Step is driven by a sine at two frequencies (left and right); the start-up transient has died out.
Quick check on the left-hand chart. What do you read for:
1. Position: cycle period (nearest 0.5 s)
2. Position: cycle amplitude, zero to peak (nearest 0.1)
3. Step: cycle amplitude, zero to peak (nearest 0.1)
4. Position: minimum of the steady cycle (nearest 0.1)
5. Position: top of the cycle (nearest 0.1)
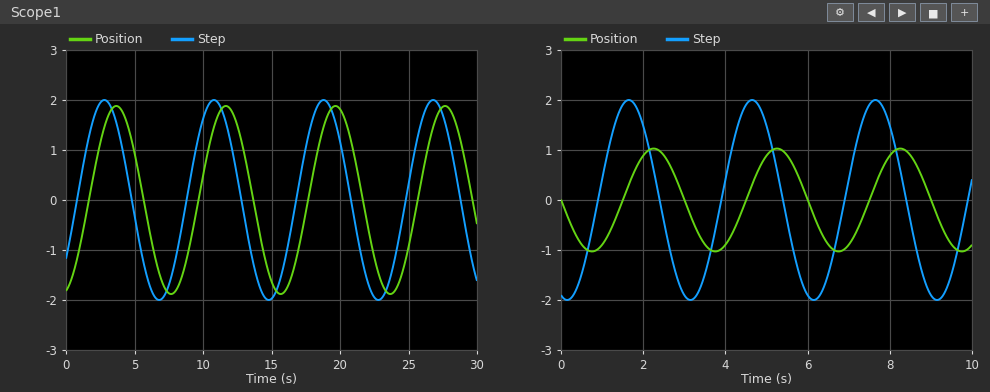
8.0 s
1.9
2.0
-1.9
1.9
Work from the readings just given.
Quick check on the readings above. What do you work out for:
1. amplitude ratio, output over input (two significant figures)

0.95
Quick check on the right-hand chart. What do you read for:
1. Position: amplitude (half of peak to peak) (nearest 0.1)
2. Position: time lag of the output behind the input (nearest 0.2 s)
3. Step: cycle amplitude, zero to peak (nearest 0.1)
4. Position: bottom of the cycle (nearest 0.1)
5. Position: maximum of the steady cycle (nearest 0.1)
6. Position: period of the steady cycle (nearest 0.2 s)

1.0
0.6 s
2.0
-1.0
1.0
3.0 s
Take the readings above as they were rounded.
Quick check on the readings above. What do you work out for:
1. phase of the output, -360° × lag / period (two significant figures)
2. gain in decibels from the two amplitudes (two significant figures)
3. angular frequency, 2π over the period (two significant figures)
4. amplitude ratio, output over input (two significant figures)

-72°
-6.0 dB
2.1 rad/s
0.50
